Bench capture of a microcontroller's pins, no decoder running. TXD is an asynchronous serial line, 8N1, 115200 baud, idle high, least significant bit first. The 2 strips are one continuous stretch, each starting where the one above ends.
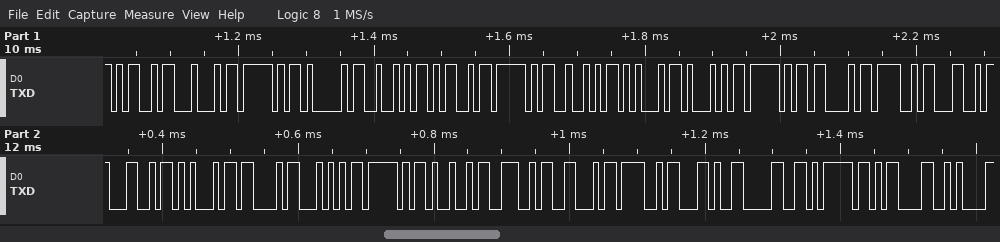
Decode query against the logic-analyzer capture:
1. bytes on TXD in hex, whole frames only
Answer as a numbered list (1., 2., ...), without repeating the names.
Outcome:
1. 4D 44 5F 41 52 4D 5F 52 45 51 5F 43 4F 4C 4C 45 43 54 5F 49 4E 46 4F 2C 30 7D 0D 0A
